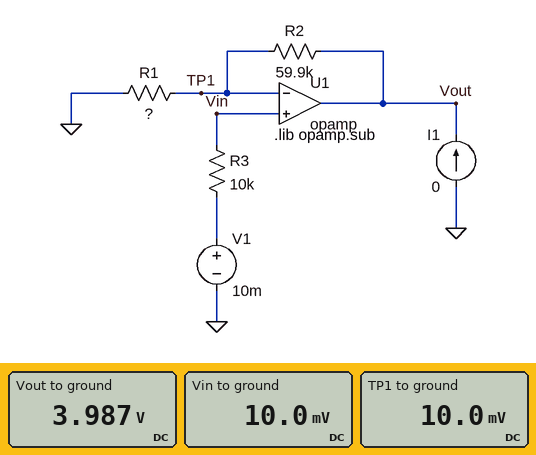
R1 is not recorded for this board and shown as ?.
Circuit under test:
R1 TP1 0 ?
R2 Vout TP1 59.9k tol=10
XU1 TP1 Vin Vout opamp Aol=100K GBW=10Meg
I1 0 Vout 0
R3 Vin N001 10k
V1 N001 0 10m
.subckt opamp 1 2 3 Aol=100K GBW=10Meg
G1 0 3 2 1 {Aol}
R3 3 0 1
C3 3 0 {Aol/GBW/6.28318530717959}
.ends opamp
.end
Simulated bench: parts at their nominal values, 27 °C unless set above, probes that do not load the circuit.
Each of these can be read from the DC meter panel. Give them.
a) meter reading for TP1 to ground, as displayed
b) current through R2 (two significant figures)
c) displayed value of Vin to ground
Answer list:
10.0 mV
66 µA
10.0 mV
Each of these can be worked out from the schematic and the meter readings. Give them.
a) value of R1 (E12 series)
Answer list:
150 Ω
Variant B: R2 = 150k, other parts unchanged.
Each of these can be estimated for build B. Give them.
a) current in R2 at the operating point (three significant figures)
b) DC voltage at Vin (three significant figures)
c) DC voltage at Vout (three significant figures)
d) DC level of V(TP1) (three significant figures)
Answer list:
66.0 µA
10.0 mV
9.91 V
9.90 mV
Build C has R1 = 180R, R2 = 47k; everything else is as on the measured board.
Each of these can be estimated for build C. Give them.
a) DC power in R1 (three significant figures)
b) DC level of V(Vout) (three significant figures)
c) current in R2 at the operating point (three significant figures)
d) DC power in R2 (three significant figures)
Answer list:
553 nW
2.61 V
55.4 µA
144 µW
